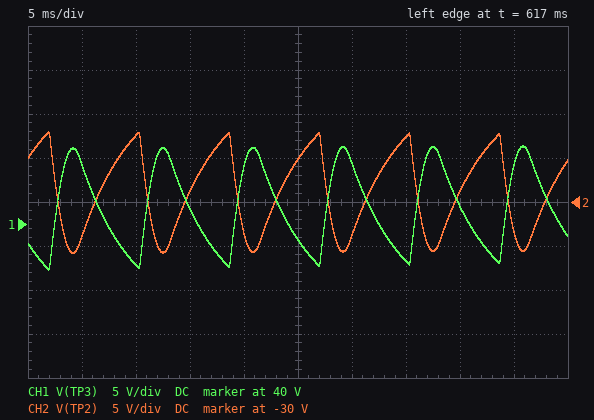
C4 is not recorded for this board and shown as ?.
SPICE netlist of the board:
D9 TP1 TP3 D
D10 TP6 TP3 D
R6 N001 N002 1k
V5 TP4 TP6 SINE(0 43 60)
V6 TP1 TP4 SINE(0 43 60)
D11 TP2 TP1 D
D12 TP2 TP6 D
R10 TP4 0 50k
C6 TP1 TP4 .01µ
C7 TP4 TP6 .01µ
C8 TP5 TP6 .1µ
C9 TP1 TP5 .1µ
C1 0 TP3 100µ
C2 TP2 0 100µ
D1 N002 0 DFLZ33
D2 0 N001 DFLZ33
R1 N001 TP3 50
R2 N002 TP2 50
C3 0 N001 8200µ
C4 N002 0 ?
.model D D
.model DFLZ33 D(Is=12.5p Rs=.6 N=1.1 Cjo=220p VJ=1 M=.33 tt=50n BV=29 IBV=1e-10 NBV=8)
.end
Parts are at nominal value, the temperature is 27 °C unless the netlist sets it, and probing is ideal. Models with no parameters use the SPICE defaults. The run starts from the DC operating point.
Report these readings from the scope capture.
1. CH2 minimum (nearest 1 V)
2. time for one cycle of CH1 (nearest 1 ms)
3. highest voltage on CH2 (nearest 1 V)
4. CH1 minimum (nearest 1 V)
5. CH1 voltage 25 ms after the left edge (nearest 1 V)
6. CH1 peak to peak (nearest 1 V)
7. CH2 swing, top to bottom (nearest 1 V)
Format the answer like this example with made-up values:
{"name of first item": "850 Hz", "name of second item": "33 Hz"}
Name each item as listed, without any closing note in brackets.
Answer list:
{"CH2 minimum": "-36 V", "time for one cycle of CH1": "8 ms", "highest voltage on CH2": "-22 V", "CH1 minimum": "35 V", "CH1 voltage 25 ms after the left edge": "38 V", "CH1 peak to peak": "14 V", "CH2 swing, top to bottom": "14 V"}
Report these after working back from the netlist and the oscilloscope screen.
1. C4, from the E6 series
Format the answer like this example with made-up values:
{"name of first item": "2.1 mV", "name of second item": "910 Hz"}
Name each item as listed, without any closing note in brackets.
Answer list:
{"C4, from the E6 series": "15 mF"}
